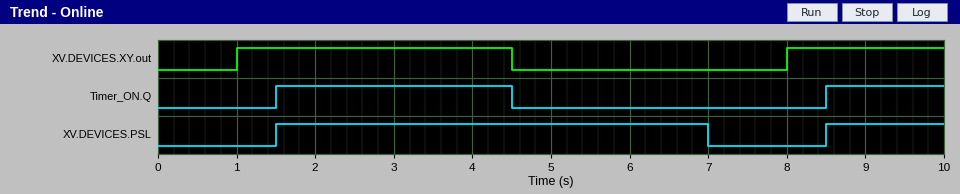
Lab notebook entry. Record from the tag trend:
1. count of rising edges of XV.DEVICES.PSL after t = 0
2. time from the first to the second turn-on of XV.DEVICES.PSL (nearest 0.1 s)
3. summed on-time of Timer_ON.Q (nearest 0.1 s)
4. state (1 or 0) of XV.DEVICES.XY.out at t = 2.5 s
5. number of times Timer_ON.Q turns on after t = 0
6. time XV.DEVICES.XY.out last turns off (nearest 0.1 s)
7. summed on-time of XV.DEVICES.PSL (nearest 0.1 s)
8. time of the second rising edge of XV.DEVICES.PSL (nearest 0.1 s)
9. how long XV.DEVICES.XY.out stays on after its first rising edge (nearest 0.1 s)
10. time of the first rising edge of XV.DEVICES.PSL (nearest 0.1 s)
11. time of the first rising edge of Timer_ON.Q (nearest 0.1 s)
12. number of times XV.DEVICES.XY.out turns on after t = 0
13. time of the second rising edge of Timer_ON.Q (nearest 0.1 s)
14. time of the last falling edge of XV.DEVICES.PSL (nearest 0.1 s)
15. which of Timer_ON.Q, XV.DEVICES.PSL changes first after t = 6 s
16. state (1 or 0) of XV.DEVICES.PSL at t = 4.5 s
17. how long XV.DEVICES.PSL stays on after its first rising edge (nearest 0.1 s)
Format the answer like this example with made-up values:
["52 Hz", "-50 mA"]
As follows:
["2", "7.0 s", "4.5 s", "1", "2", "4.5 s", "7.0 s", "8.5 s", "3.5 s", "1.5 s", "1.5 s", "2", "8.5 s", "7.0 s", "XV.DEVICES.PSL", "1", "5.5 s"]
